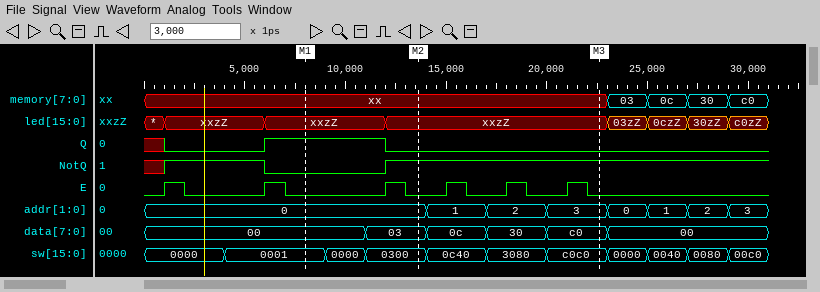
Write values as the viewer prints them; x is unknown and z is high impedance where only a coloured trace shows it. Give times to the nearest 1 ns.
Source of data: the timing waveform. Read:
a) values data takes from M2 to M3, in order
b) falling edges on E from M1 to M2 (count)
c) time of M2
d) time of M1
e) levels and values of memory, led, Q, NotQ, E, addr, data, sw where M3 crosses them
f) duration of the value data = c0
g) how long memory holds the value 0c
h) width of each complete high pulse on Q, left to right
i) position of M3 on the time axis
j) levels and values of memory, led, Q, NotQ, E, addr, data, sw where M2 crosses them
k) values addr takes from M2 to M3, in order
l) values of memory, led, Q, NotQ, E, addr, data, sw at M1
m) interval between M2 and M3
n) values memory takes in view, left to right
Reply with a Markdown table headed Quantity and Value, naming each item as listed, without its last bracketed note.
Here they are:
| Quantity | Value |
|---|---|
| values data takes from M2 to M3, in order | 03, 0c, 30, c0 |
| falling edges on E from M1 to M2 | 1 |
| time of M2 | 14 ns |
| time of M1 | 8 ns |
| levels and values of memory, led, Q, NotQ, E, addr, data, sw where M3 crosses them | memory=xx, led=xxzZ, Q=0, NotQ=1, E=0, addr=3, data=c0, sw=c0c0 |
| duration of the value data = c0 | 3 ns |
| how long memory holds the value 0c | 2 ns |
| width of each complete high pulse on Q, left to right | 6 ns |
| position of M3 on the time axis | 23 ns |
| levels and values of memory, led, Q, NotQ, E, addr, data, sw where M2 crosses them | memory=xx, led=xxzZ, Q=0, NotQ=1, E=0, addr=0, data=03, sw=0300 |
| values addr takes from M2 to M3, in order | 0, 1, 2, 3 |
| values of memory, led, Q, NotQ, E, addr, data, sw at M1 | memory=xx, led=xxzZ, Q=1, NotQ=0, E=0, addr=0, data=00, sw=0001 |
| interval between M2 and M3 | 9 ns |
| values memory takes in view, left to right | xx, 03, 0c, 30, c0 |
